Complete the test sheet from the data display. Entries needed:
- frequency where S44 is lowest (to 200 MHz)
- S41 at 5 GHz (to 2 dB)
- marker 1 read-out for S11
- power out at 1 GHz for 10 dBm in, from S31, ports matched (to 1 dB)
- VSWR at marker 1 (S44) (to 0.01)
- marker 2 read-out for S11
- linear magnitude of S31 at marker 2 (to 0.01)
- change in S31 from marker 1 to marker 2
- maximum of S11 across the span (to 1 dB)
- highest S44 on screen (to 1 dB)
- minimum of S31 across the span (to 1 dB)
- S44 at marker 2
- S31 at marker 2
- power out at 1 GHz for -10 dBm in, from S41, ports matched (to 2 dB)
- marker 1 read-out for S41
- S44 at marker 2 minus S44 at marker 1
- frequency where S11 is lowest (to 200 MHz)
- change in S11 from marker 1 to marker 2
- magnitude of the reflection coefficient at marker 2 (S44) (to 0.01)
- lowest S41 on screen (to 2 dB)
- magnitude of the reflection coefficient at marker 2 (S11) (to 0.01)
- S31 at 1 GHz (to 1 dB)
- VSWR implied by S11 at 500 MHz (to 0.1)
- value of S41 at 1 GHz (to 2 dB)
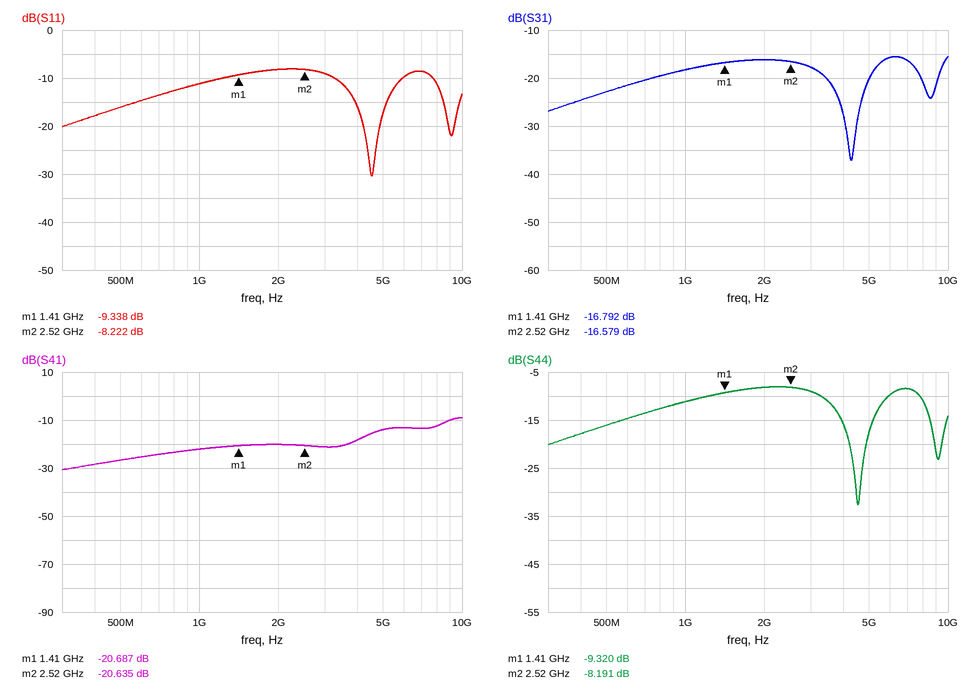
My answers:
4.6 GHz
-14 dB
-9.338 dB
-8 dBm
2.04
-8.222 dB
0.15
0.213 dB
-8 dB
-8 dB
-37 dB
-8.191 dB
-16.579 dB
-32 dBm
-20.687 dB
1.129 dB
4.6 GHz
1.116 dB
0.39
-30 dB
0.39
-18 dB
1.4
-22 dB
